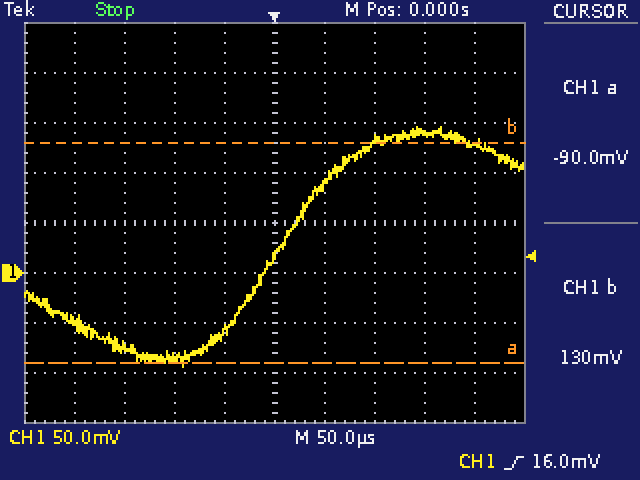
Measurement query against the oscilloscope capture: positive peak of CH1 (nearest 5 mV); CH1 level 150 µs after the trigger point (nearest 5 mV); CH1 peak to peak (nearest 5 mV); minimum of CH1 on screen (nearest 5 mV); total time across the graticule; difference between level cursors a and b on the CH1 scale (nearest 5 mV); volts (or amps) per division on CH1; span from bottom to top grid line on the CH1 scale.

145 mV
140 mV
240 mV
-95 mV
500 µs
220 mV
50 mV
400 mV
